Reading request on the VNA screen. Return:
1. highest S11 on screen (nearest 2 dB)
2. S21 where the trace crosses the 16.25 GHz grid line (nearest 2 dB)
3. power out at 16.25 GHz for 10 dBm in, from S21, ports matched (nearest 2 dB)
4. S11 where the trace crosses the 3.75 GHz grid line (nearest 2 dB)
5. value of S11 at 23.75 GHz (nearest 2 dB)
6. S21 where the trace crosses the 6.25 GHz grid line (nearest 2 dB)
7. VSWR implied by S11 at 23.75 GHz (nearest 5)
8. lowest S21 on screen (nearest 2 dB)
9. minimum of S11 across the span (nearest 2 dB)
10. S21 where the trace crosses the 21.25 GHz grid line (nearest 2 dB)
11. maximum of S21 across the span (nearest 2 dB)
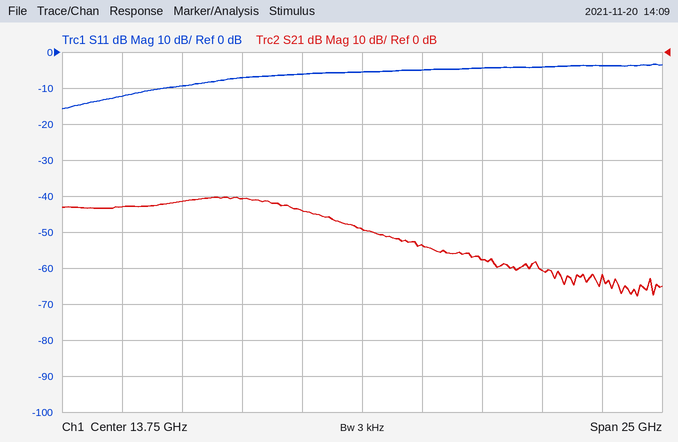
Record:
-4 dB
-54 dB
-44 dBm
-12 dB
-4 dB
-42 dB
5
-68 dB
-16 dB
-60 dB
-40 dB
